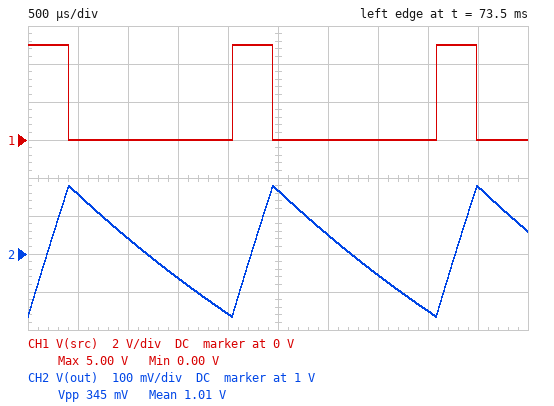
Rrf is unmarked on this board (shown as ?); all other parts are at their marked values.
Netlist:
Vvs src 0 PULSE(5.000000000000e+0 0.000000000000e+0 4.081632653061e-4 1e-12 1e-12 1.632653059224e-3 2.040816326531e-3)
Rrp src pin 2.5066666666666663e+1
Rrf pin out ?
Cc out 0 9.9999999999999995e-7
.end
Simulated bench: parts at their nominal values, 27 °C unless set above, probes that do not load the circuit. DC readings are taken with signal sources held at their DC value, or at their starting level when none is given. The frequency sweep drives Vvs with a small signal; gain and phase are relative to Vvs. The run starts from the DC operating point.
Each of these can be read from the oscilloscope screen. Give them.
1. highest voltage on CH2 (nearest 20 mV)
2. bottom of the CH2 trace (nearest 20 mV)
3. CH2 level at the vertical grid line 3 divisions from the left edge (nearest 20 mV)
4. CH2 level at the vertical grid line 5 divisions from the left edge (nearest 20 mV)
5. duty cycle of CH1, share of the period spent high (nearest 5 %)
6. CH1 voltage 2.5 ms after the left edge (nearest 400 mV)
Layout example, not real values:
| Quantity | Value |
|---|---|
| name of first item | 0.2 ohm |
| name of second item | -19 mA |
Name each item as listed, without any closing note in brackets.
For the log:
| Quantity | Value |
|---|---|
| highest voltage on CH2 | 1.18 V |
| bottom of the CH2 trace | 840 mV |
| CH2 level at the vertical grid line 3 divisions from the left edge | 940 mV |
| CH2 level at the vertical grid line 5 divisions from the left edge | 1.16 V |
| duty cycle of CH1, share of the period spent high | 20 % |
| CH1 voltage 2.5 ms after the left edge | 0 V |
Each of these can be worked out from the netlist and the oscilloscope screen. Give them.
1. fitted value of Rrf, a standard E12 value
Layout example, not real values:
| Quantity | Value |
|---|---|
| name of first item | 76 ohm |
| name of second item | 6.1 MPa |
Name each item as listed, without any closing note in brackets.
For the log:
| Quantity | Value |
|---|---|
| fitted value of Rrf, a standard E12 value | 4.7 kΩ |
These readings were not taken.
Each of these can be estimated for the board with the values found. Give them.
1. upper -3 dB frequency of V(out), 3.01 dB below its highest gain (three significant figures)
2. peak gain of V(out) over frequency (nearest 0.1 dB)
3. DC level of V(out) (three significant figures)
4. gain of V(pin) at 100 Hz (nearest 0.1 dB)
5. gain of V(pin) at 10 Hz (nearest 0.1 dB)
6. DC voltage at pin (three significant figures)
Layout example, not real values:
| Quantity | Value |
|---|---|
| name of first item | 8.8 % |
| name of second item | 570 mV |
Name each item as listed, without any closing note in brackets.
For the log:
| Quantity | Value |
|---|---|
| upper -3 dB frequency of V(out), 3.01 dB below its highest gain | 33.7 Hz |
| peak gain of V(out) over frequency | 0 dB |
| DC level of V(out) | 5.00 V |
| gain of V(pin) at 100 Hz | 0 dB |
| gain of V(pin) at 10 Hz | 0 dB |
| DC voltage at pin | 5.00 V |
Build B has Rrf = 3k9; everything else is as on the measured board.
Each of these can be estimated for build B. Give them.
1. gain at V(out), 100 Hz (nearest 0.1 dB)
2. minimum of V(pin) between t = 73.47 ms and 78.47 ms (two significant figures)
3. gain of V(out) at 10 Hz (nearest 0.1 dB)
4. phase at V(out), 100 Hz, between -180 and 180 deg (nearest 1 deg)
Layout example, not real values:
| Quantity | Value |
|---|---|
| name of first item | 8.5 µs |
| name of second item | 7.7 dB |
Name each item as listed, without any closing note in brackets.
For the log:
| Quantity | Value |
|---|---|
| gain at V(out), 100 Hz | -8.5 dB |
| minimum of V(pin) between t = 73.47 ms and 78.47 ms | 5.1 mV |
| gain of V(out) at 10 Hz | -0.3 dB |
| phase at V(out), 100 Hz, between -180 and 180 deg | -68 deg |
